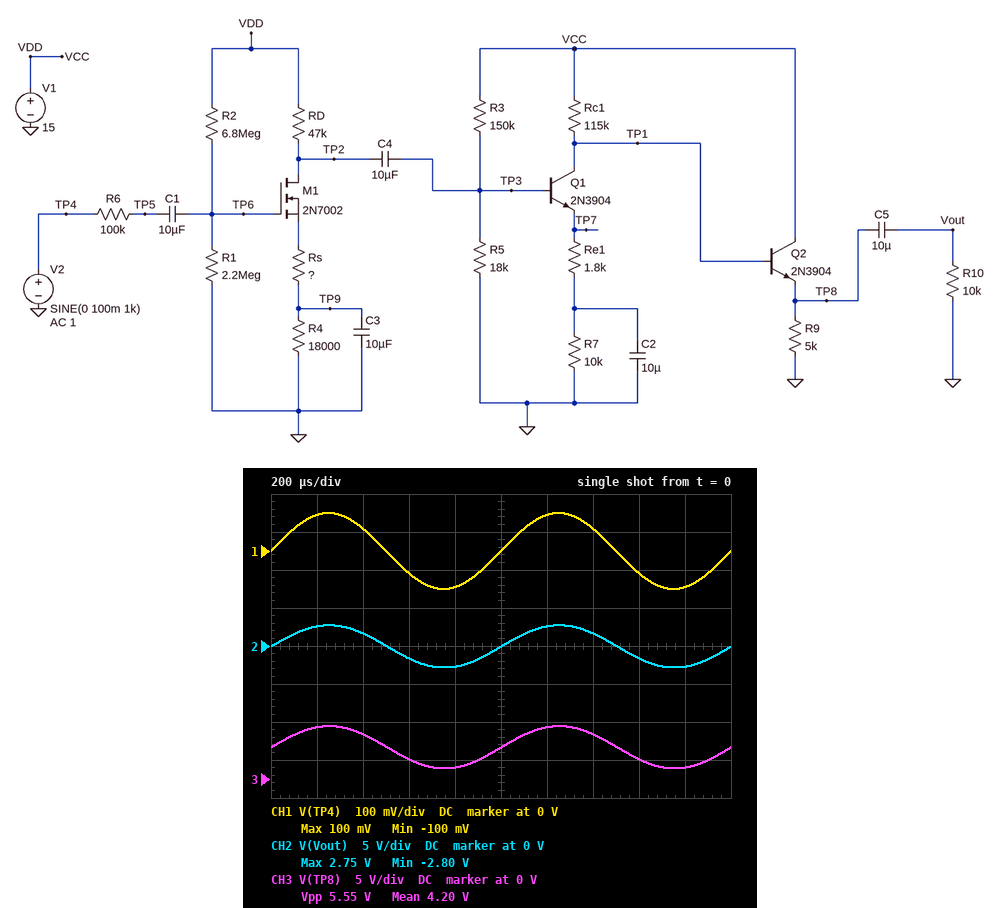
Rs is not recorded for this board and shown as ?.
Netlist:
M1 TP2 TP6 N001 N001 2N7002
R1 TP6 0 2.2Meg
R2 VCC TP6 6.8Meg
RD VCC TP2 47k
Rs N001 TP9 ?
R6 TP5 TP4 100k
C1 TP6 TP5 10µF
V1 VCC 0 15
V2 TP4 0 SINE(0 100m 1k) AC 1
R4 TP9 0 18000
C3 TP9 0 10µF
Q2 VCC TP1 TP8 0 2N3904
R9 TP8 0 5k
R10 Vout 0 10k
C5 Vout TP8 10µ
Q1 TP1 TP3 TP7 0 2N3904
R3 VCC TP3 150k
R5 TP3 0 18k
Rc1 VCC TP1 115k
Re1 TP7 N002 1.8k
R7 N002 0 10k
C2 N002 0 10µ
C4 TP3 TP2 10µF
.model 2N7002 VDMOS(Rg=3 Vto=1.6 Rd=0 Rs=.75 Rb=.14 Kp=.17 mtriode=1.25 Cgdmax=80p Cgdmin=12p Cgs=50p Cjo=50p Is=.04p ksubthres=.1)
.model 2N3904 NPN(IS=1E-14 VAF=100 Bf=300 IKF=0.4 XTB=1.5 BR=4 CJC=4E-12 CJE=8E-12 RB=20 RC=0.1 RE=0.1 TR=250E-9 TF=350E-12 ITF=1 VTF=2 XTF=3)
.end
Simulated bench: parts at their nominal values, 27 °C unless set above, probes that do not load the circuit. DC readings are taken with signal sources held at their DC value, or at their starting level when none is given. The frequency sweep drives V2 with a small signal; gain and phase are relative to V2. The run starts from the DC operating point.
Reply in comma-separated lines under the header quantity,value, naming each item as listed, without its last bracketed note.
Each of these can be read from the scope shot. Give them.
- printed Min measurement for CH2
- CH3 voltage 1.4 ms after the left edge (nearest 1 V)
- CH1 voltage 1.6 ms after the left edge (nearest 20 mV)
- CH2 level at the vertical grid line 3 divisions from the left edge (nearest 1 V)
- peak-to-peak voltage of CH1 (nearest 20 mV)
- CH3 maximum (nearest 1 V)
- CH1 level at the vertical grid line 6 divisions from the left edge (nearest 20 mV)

quantity,value
printed Min measurement for CH2,-2.80 V
CH3 voltage 1.4 ms after the left edge,6 V
CH1 voltage 1.6 ms after the left edge,-60 mV
CH2 level at the vertical grid line 3 divisions from the left edge,-2 V
peak-to-peak voltage of CH1,200 mV
CH3 maximum,7 V
CH1 level at the vertical grid line 6 divisions from the left edge,100 mV
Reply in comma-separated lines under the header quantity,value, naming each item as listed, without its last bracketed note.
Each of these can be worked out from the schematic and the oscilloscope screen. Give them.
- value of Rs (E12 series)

quantity,value
value of Rs,18 kΩ
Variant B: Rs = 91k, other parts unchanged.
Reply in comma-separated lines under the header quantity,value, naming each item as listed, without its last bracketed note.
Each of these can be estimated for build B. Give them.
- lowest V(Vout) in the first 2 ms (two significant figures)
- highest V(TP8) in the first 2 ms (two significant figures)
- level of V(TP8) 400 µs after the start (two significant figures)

quantity,value
lowest V(Vout) in the first 2 ms,-580 mV
highest V(TP8) in the first 2 ms,4.8 V
level of V(TP8) 400 µs after the start,4.6 V
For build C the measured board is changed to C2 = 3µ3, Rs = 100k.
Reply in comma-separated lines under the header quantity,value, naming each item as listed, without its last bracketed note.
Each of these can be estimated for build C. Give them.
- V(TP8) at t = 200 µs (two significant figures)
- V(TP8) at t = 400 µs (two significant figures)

quantity,value
V(TP8) at t = 200 µs,4.7 V
V(TP8) at t = 400 µs,4.5 V
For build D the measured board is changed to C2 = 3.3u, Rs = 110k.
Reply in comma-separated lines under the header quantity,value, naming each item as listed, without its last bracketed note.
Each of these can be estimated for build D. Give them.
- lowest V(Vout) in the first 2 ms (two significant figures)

quantity,value
lowest V(Vout) in the first 2 ms,-480 mV
